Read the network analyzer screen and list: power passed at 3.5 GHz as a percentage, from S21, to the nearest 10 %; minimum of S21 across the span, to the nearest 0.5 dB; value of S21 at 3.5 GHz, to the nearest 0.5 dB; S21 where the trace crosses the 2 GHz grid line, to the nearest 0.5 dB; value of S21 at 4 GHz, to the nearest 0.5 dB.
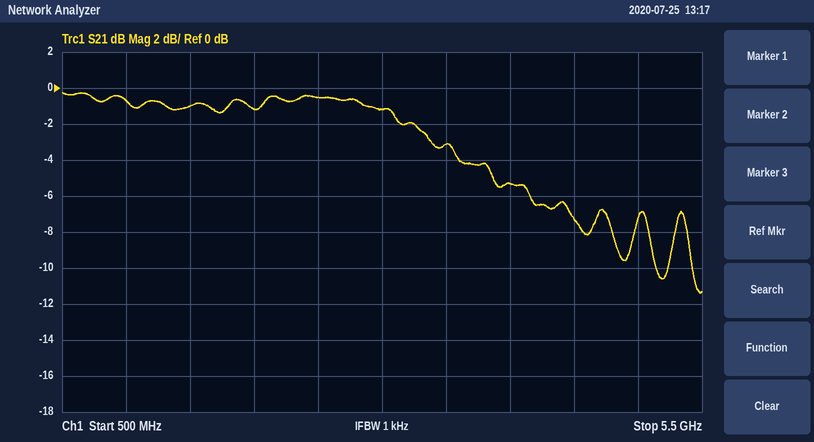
50 %
-11.5 dB
-3.0 dB
-1.0 dB
-5.5 dB
